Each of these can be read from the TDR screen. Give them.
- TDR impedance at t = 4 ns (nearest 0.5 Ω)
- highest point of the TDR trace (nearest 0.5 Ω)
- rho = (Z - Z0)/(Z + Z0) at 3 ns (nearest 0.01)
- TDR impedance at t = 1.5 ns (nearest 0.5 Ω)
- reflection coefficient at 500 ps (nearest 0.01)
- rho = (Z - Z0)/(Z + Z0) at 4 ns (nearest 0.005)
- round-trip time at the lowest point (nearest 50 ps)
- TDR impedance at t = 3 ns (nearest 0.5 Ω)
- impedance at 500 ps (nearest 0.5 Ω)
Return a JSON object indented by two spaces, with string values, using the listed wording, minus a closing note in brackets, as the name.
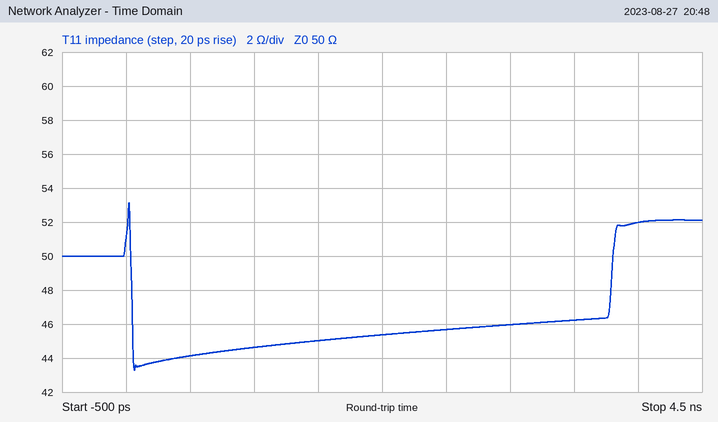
{
  "TDR impedance at t = 4 ns": "52.0 Ω",
  "highest point of the TDR trace": "53.0 Ω",
  "rho = (Z - Z0)/(Z + Z0) at 3 ns": "-0.04",
  "TDR impedance at t = 1.5 ns": "45.0 Ω",
  "reflection coefficient at 500 ps": "-0.06",
  "rho = (Z - Z0)/(Z + Z0) at 4 ns": "+0.020",
  "round-trip time at the lowest point": "50 ps",
  "TDR impedance at t = 3 ns": "46.0 Ω",
  "impedance at 500 ps": "44.0 Ω"
}
